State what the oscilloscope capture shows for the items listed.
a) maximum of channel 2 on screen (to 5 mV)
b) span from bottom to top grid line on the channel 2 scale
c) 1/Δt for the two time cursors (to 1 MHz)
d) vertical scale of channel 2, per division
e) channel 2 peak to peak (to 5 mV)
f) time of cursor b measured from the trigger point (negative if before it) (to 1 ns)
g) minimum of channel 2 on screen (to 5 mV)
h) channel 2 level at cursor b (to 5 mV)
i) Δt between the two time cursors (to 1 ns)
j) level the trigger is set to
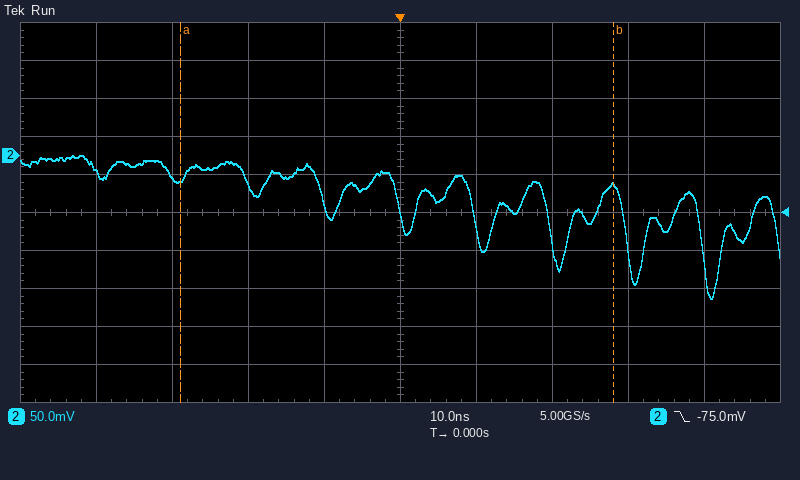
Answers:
0 mV
500 mV
18 MHz
50 mV
190 mV
+28 ns
-190 mV
-40 mV
57 ns
-75.0 mV
